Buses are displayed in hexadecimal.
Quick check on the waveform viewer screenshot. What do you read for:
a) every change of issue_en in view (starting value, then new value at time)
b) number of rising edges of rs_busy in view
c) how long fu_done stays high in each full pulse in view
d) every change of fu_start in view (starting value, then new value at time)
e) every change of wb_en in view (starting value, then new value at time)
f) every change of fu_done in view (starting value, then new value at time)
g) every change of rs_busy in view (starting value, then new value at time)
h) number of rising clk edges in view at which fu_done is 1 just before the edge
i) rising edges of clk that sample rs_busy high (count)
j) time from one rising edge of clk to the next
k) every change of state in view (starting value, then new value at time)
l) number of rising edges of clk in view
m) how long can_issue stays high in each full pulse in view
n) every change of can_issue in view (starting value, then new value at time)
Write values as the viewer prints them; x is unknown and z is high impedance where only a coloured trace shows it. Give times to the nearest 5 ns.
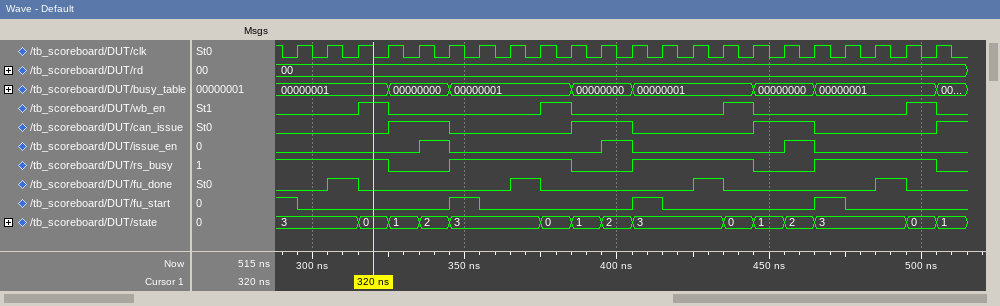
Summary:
0, 1 at 335 ns, 0 at 345 ns, 1 at 395 ns, 0 at 405 ns, 1 at 455 ns, 0 at 465 ns
3
10 ns, 10 ns, 10 ns, 10 ns
1, 0 at 295 ns, 1 at 345 ns, 0 at 355 ns, 1 at 405 ns, 0 at 415 ns, 1 at 465 ns, 0 at 475 ns
0, 1 at 315 ns, 0 at 325 ns, 1 at 375 ns, 0 at 385 ns, 1 at 435 ns, 0 at 445 ns, 1 at 495 ns, 0 at 505 ns
0, 1 at 305 ns, 0 at 315 ns, 1 at 365 ns, 0 at 375 ns, 1 at 425 ns, 0 at 435 ns, 1 at 485 ns, 0 at 495 ns
1, 0 at 325 ns, 1 at 345 ns, 0 at 385 ns, 1 at 405 ns, 0 at 445 ns, 1 at 465 ns, 0 at 505 ns
4
16
10 ns
3, 0 at 315 ns, 1 at 325 ns, 2 at 335 ns, 3 at 345 ns, 0 at 375 ns, 1 at 385 ns, 2 at 395 ns, 3 at 405 ns, 0 at 435 ns, 1 at 445 ns, 2 at 455 ns, 3 at 465 ns, 0 at 495 ns, 1 at 505 ns
22
20 ns, 20 ns, 20 ns
0, 1 at 325 ns, 0 at 345 ns, 1 at 385 ns, 0 at 405 ns, 1 at 445 ns, 0 at 465 ns, 1 at 505 ns
